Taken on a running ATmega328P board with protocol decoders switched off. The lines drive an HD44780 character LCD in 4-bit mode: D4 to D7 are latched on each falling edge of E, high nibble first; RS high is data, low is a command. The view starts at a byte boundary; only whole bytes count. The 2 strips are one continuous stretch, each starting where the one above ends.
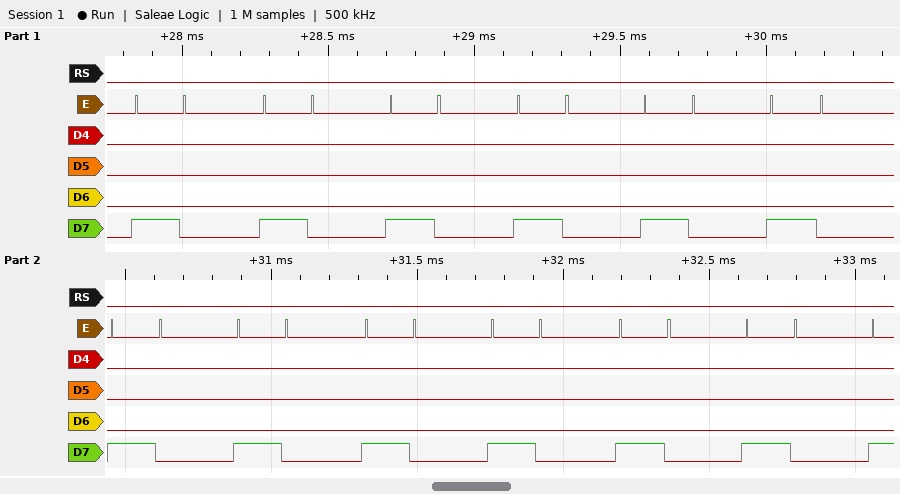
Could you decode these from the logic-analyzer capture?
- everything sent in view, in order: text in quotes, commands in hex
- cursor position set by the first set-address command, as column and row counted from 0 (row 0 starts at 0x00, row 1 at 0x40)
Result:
0x80 0x80 0x80 0x80 0x80 0x80 0x80 0x80 0x80 0x80 0x80 0x80
column 0, row 0
